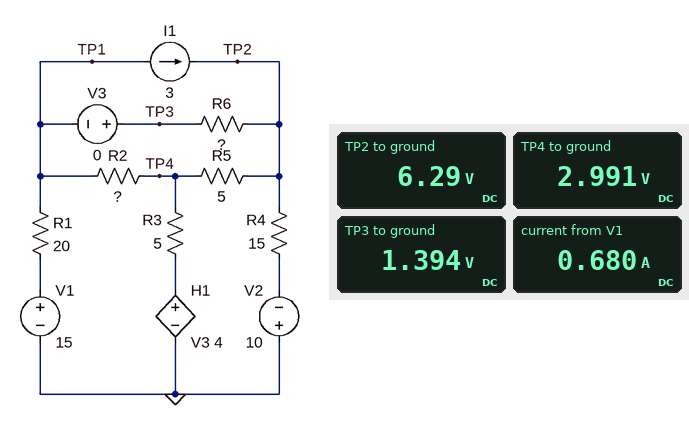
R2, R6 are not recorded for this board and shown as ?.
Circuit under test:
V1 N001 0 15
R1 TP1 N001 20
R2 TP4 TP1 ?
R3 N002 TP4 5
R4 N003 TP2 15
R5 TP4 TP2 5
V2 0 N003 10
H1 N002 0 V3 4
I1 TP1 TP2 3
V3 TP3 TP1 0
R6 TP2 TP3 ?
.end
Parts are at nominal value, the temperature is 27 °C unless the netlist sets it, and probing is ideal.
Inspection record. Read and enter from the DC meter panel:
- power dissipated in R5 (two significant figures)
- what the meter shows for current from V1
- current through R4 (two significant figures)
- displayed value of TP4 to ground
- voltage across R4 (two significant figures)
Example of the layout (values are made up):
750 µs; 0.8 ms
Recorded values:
2.2 W; 0.680 A; 1.1 A; 2.991 V; 16 V
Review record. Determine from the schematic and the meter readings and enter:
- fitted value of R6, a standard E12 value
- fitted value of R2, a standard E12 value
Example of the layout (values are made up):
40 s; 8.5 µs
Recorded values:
3.9 Ω; 1.5 Ω
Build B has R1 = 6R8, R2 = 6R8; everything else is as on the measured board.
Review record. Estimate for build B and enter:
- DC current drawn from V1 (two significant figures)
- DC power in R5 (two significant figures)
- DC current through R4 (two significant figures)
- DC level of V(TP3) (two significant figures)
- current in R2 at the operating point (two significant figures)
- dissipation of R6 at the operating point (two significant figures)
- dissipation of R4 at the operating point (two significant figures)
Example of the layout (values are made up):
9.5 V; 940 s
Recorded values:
1.6 A; 1.6 W; 1.3 A; 4.4 V; 260 mA; 5.4 W; 24 W
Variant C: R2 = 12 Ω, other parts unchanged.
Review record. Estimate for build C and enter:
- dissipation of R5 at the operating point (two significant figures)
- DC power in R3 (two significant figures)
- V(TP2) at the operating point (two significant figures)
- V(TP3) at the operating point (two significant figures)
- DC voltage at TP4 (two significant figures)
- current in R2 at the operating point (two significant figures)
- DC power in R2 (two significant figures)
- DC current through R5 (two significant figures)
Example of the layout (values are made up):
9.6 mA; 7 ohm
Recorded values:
160 mW; 480 mW; 6.3 V; -490 mV; 5.4 V; 490 mA; 2.9 W; 180 mA
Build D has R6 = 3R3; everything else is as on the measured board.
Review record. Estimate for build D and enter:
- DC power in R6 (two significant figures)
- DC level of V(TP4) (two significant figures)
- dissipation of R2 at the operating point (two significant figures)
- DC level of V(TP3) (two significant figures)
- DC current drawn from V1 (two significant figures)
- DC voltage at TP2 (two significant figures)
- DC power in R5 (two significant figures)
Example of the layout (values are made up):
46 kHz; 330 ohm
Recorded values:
5.9 W; 3.3 V; 1.5 W; 1.8 V; 660 mA; 6.2 V; 1.7 W
